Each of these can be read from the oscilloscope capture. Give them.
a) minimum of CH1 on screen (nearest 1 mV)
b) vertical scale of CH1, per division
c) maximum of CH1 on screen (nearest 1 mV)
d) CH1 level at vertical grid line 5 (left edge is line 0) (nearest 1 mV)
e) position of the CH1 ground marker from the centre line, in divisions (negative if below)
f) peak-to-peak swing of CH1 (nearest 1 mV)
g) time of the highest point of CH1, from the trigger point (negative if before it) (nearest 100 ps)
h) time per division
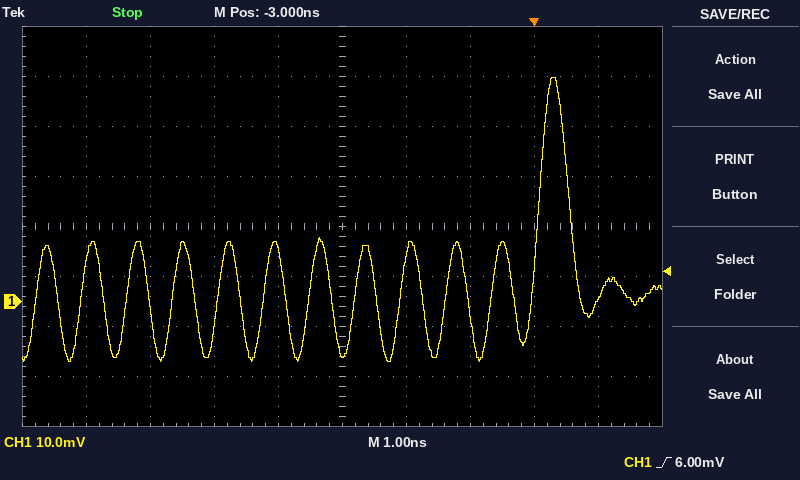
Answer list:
-12 mV
10 mV
45 mV
-10 mV
-1.5 div
57 mV
+300 ps
1 ns
